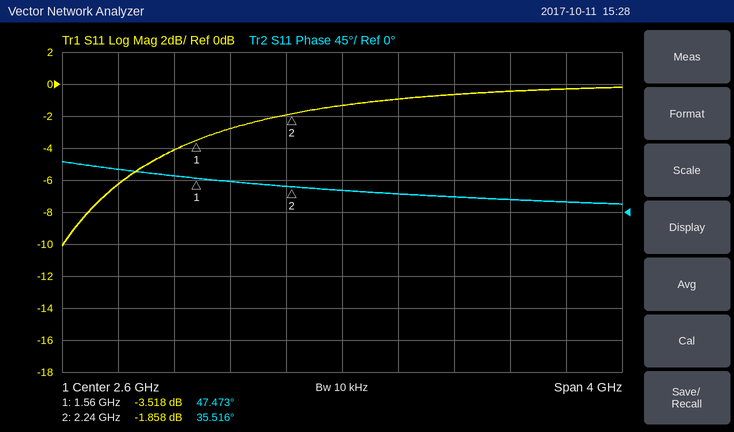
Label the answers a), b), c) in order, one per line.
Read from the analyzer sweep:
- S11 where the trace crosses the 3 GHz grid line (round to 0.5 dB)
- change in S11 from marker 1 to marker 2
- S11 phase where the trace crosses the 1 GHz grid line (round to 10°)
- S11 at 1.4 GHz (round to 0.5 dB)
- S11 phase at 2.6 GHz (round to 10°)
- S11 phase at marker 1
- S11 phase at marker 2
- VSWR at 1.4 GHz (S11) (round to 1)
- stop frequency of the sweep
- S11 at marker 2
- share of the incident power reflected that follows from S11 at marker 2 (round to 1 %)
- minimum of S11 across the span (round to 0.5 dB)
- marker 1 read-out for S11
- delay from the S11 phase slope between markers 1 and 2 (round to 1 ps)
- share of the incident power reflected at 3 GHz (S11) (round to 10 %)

a) -1.0 dB
b) 1.660 dB
c) 60°
d) -4.0 dB
e) 30°
f) 47.473°
g) 35.516°
h) 4
i) 4.6 GHz
j) -1.858 dB
k) 65 %
l) -10.0 dB
m) -3.518 dB
n) 49 ps
o) 80 %
